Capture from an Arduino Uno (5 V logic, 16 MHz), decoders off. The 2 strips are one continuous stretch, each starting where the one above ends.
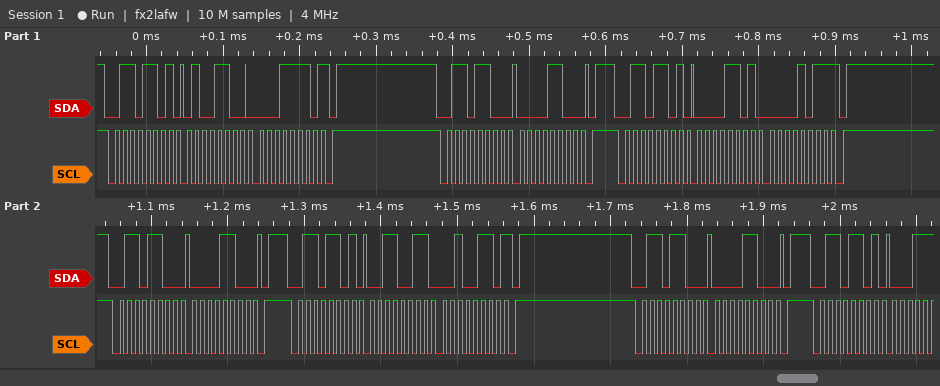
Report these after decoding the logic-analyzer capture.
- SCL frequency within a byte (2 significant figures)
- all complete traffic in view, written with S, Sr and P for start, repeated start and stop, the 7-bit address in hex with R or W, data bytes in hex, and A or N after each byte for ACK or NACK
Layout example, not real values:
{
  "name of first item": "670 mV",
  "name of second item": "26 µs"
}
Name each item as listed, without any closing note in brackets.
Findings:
{
  "SCL frequency within a byte": "100 kHz",
  "all complete traffic in view, written with S, Sr and P for start, repeated start and stop, the 7-bit address in hex with R or W, data bytes in hex, and A or N after each byte for ACK or NACK": "S 36R A 4C A 1E N P S 36W A 0C A P S 36R A 0D A 0B N P S 36W A 0C A P S 36R A 33 A 26 N P S 36W A 0C A P S 36R A"
}
